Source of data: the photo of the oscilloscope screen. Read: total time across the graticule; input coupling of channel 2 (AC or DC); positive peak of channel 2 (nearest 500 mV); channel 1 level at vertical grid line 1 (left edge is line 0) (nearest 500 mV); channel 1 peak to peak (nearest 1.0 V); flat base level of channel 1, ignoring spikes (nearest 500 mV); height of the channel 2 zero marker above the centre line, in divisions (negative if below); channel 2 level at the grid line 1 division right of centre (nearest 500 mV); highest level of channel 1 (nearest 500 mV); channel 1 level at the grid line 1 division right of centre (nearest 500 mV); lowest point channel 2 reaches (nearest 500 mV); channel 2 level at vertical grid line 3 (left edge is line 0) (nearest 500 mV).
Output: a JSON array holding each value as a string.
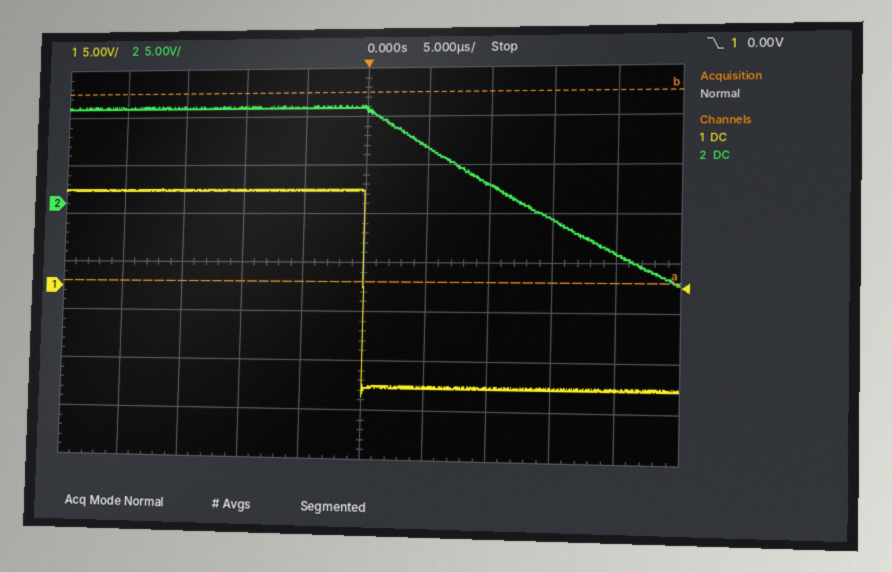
["50 µs", "DC", "10.0 V", "10.0 V", "21.0 V", "-10.0 V", "+1.2 div", "6.0 V", "10.0 V", "-10.0 V", "-8.0 V", "10.0 V"]
